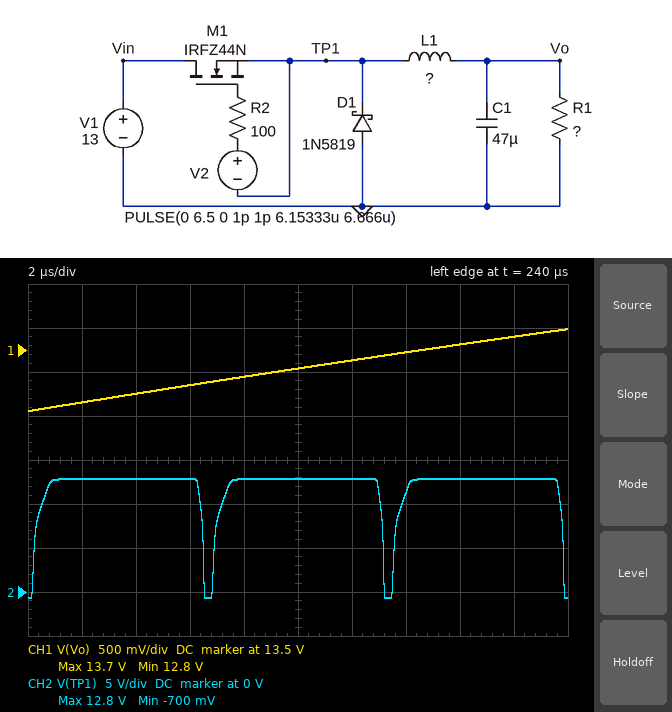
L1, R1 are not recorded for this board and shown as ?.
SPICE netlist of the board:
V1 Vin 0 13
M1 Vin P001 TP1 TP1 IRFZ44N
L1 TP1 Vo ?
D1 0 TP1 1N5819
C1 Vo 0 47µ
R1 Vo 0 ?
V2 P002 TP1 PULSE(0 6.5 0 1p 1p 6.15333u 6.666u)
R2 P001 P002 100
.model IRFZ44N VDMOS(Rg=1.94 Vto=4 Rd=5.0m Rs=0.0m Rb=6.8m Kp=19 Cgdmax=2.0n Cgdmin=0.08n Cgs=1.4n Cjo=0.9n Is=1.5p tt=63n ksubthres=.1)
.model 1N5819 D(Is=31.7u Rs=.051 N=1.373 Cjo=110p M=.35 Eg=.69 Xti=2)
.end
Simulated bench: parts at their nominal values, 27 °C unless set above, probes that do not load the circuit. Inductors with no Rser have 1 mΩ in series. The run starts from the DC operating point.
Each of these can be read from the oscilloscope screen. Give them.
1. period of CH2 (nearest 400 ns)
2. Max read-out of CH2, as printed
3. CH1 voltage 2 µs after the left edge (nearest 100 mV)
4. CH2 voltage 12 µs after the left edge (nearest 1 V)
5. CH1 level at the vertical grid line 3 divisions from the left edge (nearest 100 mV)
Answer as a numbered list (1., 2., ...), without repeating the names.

1. 6.8 µs
2. 12.8 V
3. 12.9 V
4. 13 V
5. 13.1 V
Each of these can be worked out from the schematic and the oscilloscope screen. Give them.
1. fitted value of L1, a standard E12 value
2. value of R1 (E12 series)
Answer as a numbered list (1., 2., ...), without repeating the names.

1. 270 µH
2. 3.9 Ω
